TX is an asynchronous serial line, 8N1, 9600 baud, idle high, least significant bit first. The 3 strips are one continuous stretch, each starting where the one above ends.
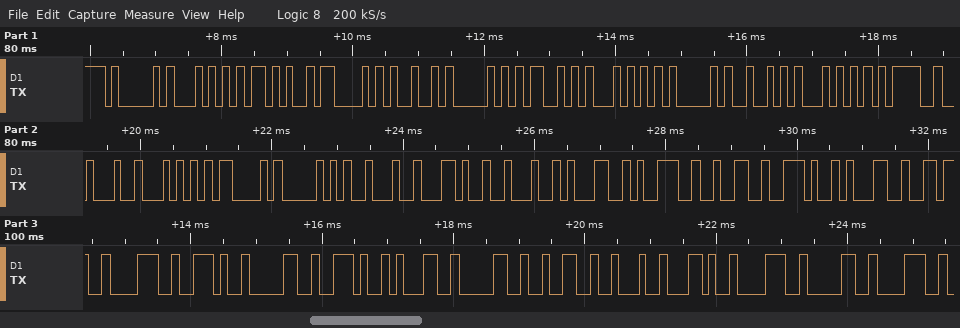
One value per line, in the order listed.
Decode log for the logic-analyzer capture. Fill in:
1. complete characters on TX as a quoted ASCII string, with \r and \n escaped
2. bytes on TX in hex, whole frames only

"AT+CIPSTART=\"TCP\",\"192.168.0.102\",808"
41 54 2B 43 49 50 53 54 41 52 54 3D 22 54 43 50 22 2C 22 31 39 32 2E 31 36 38 2E 30 2E 31 30 32 22 2C 38 30 38
